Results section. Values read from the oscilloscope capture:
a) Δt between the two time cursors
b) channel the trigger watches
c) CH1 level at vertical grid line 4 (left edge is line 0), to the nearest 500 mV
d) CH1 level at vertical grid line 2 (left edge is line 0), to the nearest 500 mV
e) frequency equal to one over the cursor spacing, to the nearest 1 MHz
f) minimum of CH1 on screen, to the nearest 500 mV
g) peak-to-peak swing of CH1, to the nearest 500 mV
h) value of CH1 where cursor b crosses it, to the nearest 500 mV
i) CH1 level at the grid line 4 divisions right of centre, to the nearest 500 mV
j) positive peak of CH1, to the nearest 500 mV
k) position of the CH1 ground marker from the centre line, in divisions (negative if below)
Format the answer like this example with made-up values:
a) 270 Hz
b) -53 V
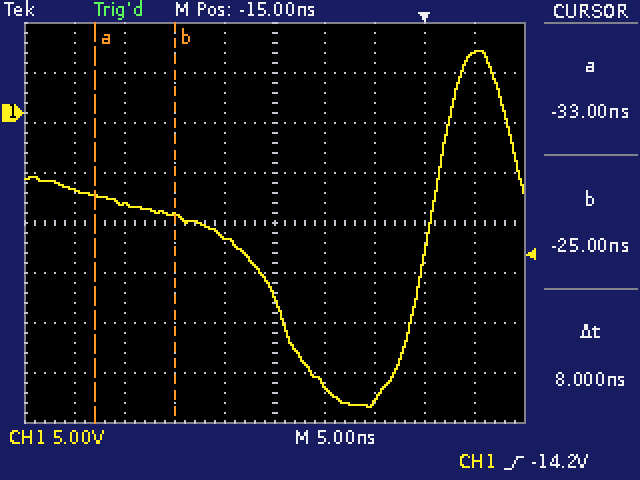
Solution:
a) 8 ns
b) CH1
c) -12.5 V
d) -9.0 V
e) 125 MHz
f) -29.5 V
g) 35.5 V
h) -10.5 V
i) 6.0 V
j) 6.0 V
k) +2.2 div
